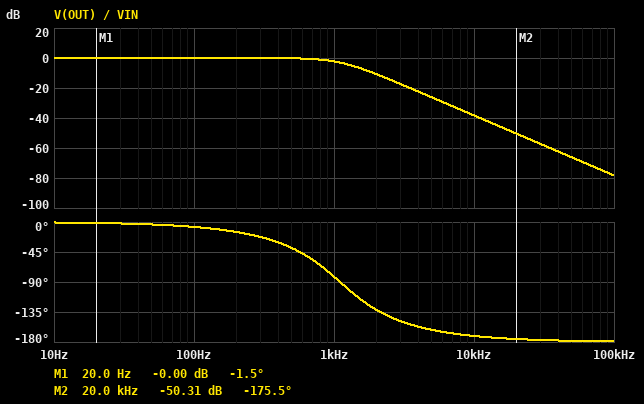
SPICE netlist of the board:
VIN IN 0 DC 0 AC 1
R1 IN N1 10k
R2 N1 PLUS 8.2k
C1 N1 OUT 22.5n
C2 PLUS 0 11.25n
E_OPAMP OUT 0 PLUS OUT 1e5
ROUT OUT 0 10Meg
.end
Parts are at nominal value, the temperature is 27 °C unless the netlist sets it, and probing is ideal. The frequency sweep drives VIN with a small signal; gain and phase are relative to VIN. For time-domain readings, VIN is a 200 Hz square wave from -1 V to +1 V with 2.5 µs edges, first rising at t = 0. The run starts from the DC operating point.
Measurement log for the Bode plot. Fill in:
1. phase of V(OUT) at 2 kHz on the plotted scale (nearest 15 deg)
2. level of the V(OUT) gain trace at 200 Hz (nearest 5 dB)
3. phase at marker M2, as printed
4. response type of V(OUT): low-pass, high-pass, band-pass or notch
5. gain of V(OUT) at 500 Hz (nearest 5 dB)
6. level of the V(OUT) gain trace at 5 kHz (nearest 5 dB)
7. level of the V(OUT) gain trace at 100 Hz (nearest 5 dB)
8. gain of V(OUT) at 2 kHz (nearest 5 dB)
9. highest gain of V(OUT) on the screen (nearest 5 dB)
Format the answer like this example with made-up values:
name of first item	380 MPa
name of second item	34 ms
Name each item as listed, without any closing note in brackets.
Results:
phase of V(OUT) at 2 kHz on the plotted scale	-135 deg
level of the V(OUT) gain trace at 200 Hz	0 dB
phase at marker M2, as printed	-175.5 deg
response type of V(OUT): low-pass, high-pass, band-pass or notch	low-pass
gain of V(OUT) at 500 Hz	0 dB
level of the V(OUT) gain trace at 5 kHz	-25 dB
level of the V(OUT) gain trace at 100 Hz	0 dB
gain of V(OUT) at 2 kHz	-10 dB
highest gain of V(OUT) on the screen	0 dB
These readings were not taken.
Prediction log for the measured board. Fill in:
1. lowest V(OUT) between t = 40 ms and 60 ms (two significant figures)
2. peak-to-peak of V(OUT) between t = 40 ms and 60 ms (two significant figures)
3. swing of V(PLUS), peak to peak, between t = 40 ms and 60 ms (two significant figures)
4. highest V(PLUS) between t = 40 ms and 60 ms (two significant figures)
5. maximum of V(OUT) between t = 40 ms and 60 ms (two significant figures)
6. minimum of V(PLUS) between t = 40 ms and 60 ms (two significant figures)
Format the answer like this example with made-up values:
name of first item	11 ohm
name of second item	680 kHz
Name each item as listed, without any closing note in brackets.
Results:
lowest V(OUT) between t = 40 ms and 60 ms	-1.1 V
peak-to-peak of V(OUT) between t = 40 ms and 60 ms	2.2 V
swing of V(PLUS), peak to peak, between t = 40 ms and 60 ms	2.2 V
highest V(PLUS) between t = 40 ms and 60 ms	1.1 V
maximum of V(OUT) between t = 40 ms and 60 ms	1.1 V
minimum of V(PLUS) between t = 40 ms and 60 ms	-1.1 V
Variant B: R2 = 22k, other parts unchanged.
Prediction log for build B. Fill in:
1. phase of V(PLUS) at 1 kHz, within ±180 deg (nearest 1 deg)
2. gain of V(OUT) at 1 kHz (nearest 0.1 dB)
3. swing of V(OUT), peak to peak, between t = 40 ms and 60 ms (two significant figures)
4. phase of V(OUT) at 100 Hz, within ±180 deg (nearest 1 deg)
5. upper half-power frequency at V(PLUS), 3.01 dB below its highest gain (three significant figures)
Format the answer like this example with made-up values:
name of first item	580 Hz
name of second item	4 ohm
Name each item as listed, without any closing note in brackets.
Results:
phase of V(PLUS) at 1 kHz, within ±180 deg	-118 deg
gain of V(OUT) at 1 kHz	-8.2 dB
swing of V(OUT), peak to peak, between t = 40 ms and 60 ms	2.1 V
phase of V(OUT) at 100 Hz, within ±180 deg	-13 deg
upper half-power frequency at V(PLUS), 3.01 dB below its highest gain	622 Hz
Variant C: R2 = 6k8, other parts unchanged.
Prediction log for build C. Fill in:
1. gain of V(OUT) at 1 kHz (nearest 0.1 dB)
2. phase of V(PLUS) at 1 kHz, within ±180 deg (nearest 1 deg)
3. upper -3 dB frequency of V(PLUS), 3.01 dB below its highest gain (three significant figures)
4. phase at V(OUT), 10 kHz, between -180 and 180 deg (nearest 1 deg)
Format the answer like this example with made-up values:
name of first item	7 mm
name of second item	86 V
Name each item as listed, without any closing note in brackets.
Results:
gain of V(OUT) at 1 kHz	-1.8 dB
phase of V(PLUS) at 1 kHz, within ±180 deg	-75 deg
upper -3 dB frequency of V(PLUS), 3.01 dB below its highest gain	1.19 kHz
phase at V(OUT), 10 kHz, between -180 and 180 deg	-170 deg
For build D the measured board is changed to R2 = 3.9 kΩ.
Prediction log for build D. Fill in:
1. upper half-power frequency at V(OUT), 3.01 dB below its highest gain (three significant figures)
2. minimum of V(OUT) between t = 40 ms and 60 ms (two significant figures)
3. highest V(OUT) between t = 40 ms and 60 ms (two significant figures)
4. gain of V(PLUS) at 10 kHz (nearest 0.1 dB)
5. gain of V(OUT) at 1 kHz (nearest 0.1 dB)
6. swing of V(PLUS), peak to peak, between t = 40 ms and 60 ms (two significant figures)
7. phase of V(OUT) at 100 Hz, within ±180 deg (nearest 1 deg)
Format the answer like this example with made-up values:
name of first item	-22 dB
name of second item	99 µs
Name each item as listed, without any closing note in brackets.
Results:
upper half-power frequency at V(OUT), 3.01 dB below its highest gain	1.42 kHz
minimum of V(OUT) between t = 40 ms and 60 ms	-1.0 V
highest V(OUT) between t = 40 ms and 60 ms	1.0 V
gain of V(PLUS) at 10 kHz	-31.9 dB
gain of V(OUT) at 1 kHz	-1.3 dB
swing of V(PLUS), peak to peak, between t = 40 ms and 60 ms	2.1 V
phase of V(OUT) at 100 Hz, within ±180 deg	-6 deg
